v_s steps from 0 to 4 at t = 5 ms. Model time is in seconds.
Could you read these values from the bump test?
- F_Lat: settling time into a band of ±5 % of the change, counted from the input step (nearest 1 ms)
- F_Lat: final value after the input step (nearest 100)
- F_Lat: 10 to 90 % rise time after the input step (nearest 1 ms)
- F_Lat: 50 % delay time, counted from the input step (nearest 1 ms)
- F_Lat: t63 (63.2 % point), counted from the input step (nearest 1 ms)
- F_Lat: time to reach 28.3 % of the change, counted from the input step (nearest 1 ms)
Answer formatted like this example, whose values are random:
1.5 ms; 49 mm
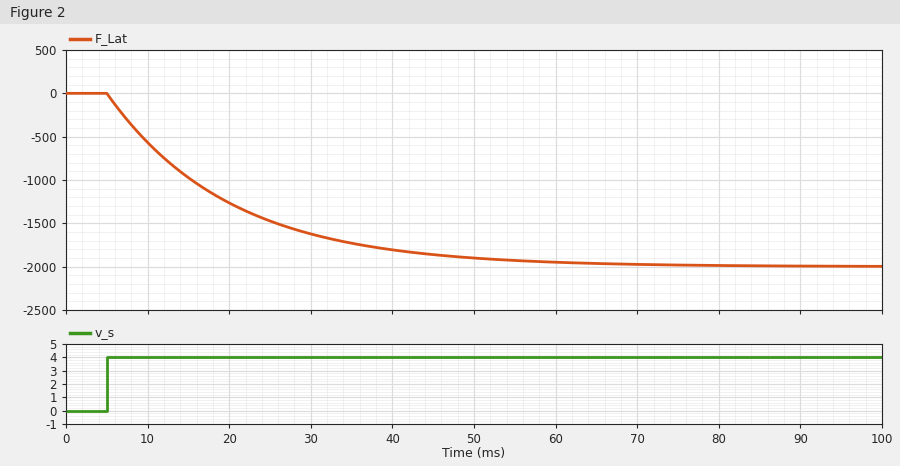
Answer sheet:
45 ms; -2000; 33 ms; 10 ms; 15 ms; 5 ms
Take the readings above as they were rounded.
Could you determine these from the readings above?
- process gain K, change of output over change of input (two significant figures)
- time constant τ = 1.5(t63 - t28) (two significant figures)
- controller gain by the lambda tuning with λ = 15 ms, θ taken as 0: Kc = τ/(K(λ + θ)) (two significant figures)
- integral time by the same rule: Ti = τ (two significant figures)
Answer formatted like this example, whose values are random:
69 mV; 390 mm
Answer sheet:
-500; 15 ms; -0.0020; 15 ms
